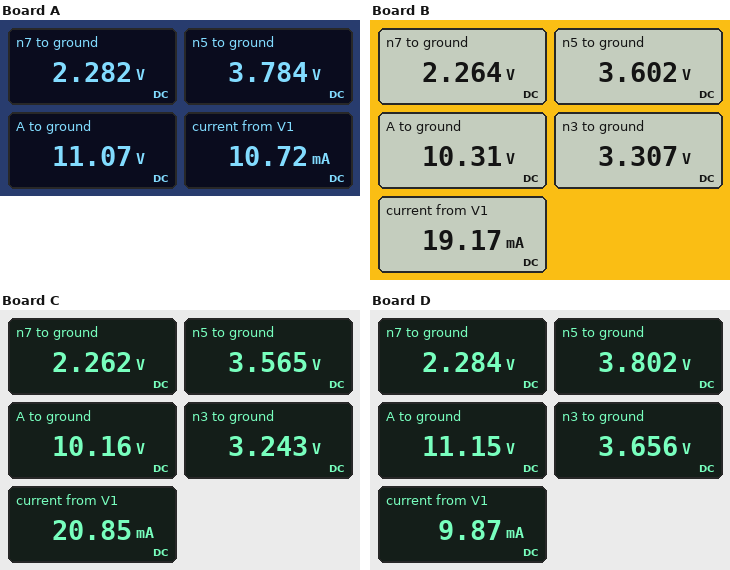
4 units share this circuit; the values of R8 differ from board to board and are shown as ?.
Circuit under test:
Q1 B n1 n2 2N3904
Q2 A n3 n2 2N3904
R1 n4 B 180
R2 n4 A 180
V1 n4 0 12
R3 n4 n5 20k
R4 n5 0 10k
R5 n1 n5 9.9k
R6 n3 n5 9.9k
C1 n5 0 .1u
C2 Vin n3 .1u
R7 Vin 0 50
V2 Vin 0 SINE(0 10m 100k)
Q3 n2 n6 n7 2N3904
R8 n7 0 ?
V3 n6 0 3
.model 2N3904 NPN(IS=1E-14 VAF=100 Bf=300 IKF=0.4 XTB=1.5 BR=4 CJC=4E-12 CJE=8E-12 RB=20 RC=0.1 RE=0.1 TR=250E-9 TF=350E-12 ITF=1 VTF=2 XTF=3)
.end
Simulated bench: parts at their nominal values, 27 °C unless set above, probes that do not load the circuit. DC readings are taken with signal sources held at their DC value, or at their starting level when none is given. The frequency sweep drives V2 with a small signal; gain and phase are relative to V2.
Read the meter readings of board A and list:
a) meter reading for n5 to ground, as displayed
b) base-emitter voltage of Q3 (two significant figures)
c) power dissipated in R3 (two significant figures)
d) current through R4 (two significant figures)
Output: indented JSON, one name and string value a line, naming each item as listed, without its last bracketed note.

{
  "meter reading for n5 to ground, as displayed": "3.784 V",
  "base-emitter voltage of Q3": "720 mV",
  "power dissipated in R3": "3.4 mW",
  "current through R4": "380 µA"
}
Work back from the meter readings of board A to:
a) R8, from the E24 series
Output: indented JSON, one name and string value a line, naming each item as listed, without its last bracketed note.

{
  "R8, from the E24 series": "220 Ω"
}
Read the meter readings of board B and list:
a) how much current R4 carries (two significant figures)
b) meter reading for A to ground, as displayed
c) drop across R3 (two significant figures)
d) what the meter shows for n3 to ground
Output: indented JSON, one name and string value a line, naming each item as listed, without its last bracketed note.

{
  "how much current R4 carries": "360 µA",
  "meter reading for A to ground, as displayed": "10.31 V",
  "drop across R3": "8.4 V",
  "what the meter shows for n3 to ground": "3.307 V"
}
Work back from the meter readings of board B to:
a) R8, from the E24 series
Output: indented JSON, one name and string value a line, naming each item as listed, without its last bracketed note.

{
  "R8, from the E24 series": "120 Ω"
}
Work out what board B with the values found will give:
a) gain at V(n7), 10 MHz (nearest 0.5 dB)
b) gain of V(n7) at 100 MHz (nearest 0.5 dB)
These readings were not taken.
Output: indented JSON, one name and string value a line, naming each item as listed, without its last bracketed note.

{
  "gain at V(n7), 10 MHz": "-43.0 dB",
  "gain of V(n7) at 100 MHz": "-23.0 dB"
}
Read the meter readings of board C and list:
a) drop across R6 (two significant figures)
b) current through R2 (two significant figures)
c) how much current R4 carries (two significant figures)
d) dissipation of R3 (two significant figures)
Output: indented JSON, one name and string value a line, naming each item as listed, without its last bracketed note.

{
  "drop across R6": "320 mV",
  "current through R2": "10 mA",
  "how much current R4 carries": "360 µA",
  "dissipation of R3": "3.6 mW"
}
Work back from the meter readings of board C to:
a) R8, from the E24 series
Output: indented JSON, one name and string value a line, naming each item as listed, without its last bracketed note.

{
  "R8, from the E24 series": "110 Ω"
}
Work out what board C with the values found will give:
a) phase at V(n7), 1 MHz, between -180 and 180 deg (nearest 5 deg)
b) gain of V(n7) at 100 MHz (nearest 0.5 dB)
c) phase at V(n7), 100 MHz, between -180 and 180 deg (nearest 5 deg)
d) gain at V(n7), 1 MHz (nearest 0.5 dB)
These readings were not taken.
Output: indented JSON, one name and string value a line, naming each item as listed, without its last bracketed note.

{
  "phase at V(n7), 1 MHz, between -180 and 180 deg": "75 deg",
  "gain of V(n7) at 100 MHz": "-15.0 dB",
  "phase at V(n7), 100 MHz, between -180 and 180 deg": "70 deg",
  "gain at V(n7), 1 MHz": "-55.0 dB"
}
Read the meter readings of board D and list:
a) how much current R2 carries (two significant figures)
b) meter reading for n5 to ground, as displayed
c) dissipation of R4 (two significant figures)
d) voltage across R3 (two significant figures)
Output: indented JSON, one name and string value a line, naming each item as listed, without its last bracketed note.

{
  "how much current R2 carries": "4.7 mA",
  "meter reading for n5 to ground, as displayed": "3.802 V",
  "dissipation of R4": "1.4 mW",
  "voltage across R3": "8.2 V"
}
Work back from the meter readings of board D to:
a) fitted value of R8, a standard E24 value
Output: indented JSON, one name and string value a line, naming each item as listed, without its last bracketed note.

{
  "fitted value of R8, a standard E24 value": "240 Ω"
}
